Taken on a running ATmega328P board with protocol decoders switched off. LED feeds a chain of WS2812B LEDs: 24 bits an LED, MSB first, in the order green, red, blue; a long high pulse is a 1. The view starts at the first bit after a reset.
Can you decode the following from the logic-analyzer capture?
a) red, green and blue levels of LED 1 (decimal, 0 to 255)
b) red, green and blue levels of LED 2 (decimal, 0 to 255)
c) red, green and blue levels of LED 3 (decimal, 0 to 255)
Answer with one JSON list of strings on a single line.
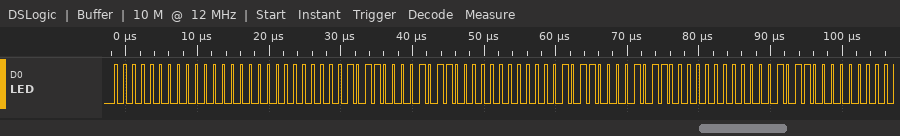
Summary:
["0, 0, 0", "44, 44, 0", "44, 44, 0"]
